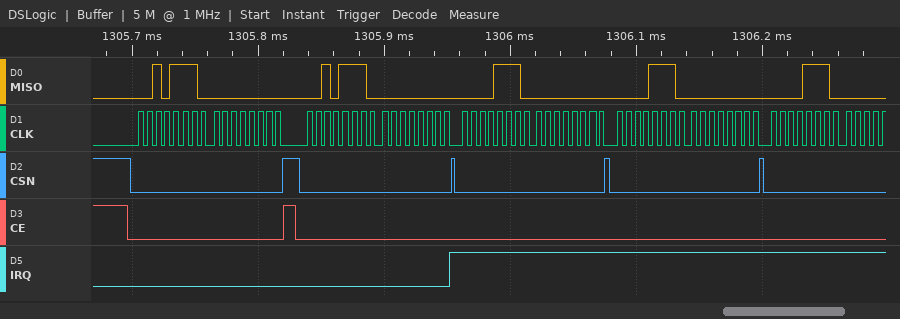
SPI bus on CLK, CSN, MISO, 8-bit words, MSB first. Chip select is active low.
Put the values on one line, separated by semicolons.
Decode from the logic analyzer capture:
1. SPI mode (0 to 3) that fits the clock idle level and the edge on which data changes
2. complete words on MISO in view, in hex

0; 2E, 00, 2E, 00, 0E, 00, 0E, 00, 0E
